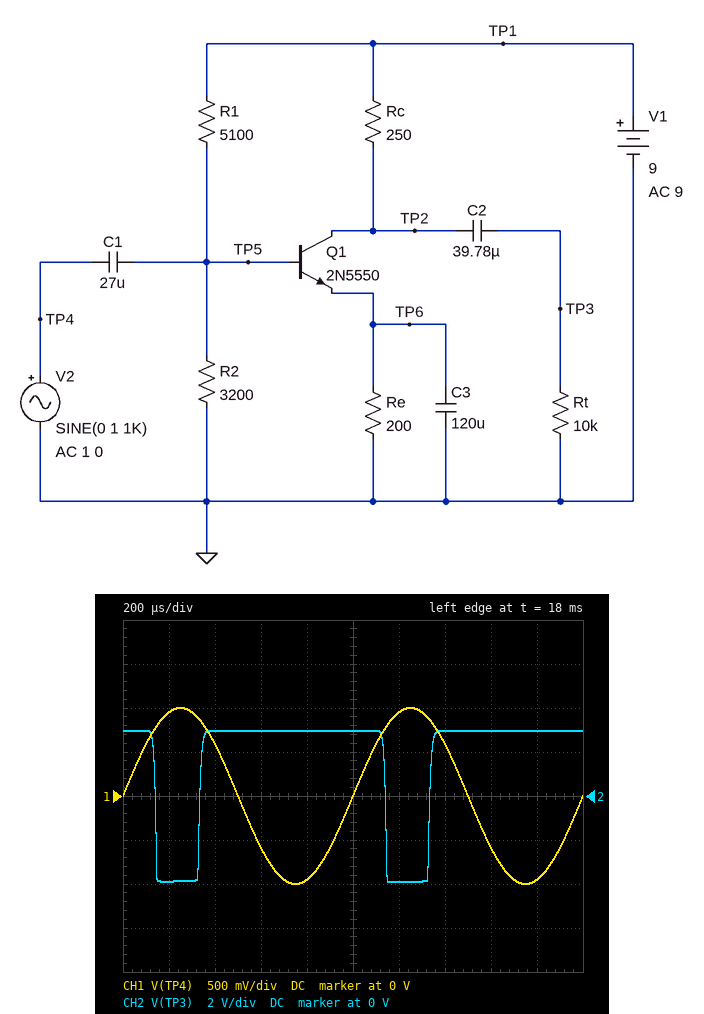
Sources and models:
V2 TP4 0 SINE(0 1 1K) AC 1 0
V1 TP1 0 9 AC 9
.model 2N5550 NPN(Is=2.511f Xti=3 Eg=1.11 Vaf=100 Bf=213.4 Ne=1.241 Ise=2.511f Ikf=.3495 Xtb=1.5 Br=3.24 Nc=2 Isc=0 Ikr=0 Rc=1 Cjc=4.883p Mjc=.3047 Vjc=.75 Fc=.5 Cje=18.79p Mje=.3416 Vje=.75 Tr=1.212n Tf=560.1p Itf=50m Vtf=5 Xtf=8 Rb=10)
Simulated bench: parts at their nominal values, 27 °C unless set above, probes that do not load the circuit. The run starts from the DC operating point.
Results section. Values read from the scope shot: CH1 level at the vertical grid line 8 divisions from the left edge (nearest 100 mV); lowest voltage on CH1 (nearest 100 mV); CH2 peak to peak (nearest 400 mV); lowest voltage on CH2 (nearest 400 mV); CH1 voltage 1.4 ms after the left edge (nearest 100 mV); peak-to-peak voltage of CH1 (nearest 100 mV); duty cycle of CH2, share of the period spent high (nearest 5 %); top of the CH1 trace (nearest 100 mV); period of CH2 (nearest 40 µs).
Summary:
-600 mV
-1.0 V
6.8 V
-4.0 V
600 mV
2.0 V
80 %
1.0 V
1.00 ms
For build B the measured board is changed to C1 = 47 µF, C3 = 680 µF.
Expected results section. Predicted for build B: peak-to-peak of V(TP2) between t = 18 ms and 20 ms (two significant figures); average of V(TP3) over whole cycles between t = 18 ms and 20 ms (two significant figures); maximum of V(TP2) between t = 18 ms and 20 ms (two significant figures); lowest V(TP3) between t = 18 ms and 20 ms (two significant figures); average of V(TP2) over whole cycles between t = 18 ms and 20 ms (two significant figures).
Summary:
6.5 V
1.8 V
8.9 V
-3.5 V
7.8 V
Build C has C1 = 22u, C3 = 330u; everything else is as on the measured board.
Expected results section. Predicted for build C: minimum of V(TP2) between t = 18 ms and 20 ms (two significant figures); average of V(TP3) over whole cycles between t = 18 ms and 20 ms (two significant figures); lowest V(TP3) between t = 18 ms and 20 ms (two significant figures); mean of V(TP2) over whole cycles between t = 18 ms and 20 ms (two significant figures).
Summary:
2.3 V
1.8 V
-3.7 V
7.8 V
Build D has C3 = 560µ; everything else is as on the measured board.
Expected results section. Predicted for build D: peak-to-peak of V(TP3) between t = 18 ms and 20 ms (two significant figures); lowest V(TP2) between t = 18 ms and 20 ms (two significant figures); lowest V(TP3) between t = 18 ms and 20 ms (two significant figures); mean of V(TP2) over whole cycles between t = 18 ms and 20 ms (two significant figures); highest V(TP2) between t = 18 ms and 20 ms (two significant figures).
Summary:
6.5 V
2.4 V
-3.6 V
7.8 V
8.9 V
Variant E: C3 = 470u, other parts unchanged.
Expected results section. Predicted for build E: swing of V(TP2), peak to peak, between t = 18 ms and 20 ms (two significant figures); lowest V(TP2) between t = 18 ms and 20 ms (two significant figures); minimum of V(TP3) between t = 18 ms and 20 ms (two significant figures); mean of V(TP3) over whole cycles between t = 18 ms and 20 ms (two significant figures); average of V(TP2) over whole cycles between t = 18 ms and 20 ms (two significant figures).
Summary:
6.6 V
2.4 V
-3.6 V
1.8 V
7.8 V
